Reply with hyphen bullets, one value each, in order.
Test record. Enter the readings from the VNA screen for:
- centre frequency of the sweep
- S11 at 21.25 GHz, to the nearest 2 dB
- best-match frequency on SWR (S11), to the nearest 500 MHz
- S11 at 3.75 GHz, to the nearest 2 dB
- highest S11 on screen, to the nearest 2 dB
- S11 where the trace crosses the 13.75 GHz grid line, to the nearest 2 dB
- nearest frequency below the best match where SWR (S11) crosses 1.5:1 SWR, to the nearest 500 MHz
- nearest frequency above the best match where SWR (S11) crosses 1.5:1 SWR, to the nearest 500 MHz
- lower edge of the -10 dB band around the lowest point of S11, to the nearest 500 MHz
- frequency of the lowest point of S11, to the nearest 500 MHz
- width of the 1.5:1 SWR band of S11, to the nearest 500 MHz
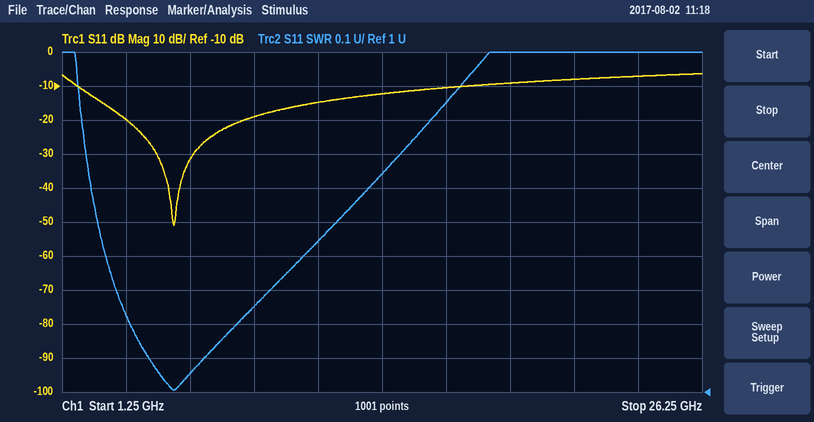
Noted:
- 13.75 GHz
- -8 dB
- 5.5 GHz
- -20 dB
- -6 dB
- -12 dB
- 2.5 GHz
- 12.0 GHz
- 2.0 GHz
- 5.5 GHz
- 9.5 GHz
